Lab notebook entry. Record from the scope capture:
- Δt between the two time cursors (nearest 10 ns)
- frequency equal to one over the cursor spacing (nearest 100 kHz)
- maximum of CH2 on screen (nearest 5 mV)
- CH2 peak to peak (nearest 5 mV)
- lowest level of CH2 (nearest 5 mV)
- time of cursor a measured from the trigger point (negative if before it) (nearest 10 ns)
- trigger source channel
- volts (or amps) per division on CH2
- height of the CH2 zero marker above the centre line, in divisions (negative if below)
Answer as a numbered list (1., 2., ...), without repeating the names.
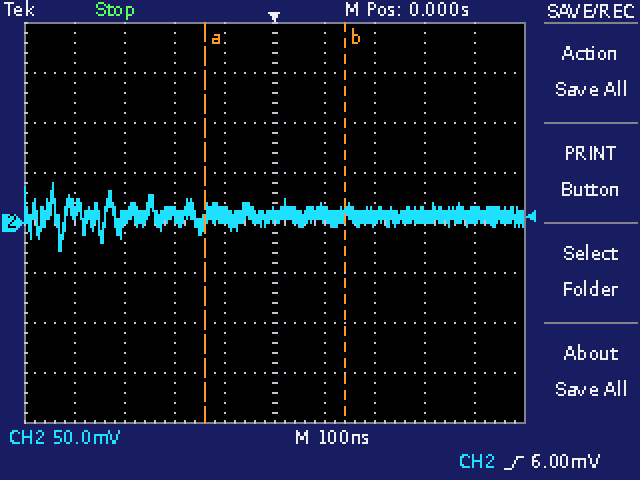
1. 280 ns
2. 3.6 MHz
3. 40 mV
4. 70 mV
5. -30 mV
6. -140 ns
7. CH2
8. 50 mV
9. 0.0 div
